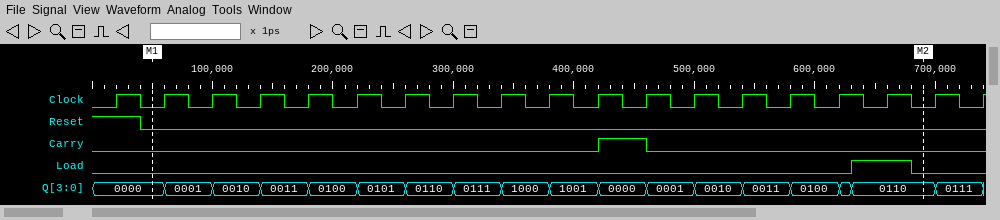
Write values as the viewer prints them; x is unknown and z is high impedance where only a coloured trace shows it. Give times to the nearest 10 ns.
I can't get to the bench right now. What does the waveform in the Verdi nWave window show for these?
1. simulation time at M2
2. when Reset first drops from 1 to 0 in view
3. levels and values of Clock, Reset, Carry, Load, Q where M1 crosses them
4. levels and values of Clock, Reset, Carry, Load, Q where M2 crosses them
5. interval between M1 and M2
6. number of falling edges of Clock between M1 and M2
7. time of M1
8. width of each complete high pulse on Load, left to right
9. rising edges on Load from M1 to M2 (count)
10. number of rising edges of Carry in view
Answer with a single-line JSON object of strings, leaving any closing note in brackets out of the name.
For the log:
{"simulation time at M2": "690 ns", "when Reset first drops from 1 to 0 in view": "40 ns", "levels and values of Clock, Reset, Carry, Load, Q where M1 crosses them": "Clock=0, Reset=0, Carry=0, Load=0, Q=0000", "levels and values of Clock, Reset, Carry, Load, Q where M2 crosses them": "Clock=0, Reset=0, Carry=0, Load=0, Q=0110", "interval between M1 and M2": "640 ns", "number of falling edges of Clock between M1 and M2": "16", "time of M1": "50 ns", "width of each complete high pulse on Load, left to right": "50 ns", "rising edges on Load from M1 to M2": "1", "number of rising edges of Carry in view": "1"}
